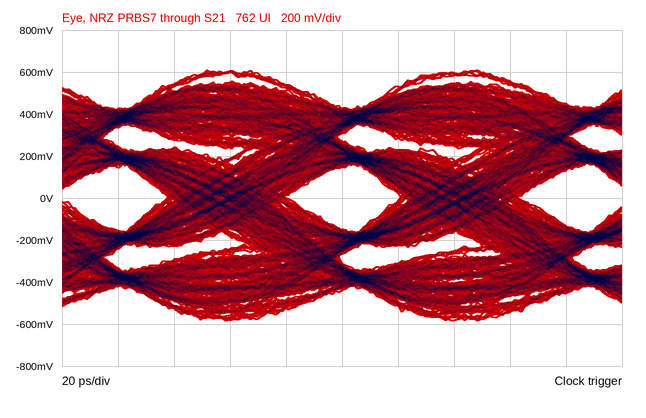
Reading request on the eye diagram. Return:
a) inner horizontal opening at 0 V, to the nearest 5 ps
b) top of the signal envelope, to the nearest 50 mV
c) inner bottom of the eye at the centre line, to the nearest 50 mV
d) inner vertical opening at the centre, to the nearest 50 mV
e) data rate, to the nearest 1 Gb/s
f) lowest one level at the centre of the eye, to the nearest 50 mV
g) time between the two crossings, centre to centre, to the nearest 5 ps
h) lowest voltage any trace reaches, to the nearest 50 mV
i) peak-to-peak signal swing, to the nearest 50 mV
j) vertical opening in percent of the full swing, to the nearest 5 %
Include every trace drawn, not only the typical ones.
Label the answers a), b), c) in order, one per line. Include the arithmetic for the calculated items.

a) 40 ps
b) 600 mV
c) -150 mV
d) 300 mV
e) 12 Gb/s
f) 150 mV
g) 85 ps
h) -600 mV
i) 1.20 V
j) 300 mV / 1.20 V ≈ 25 %
